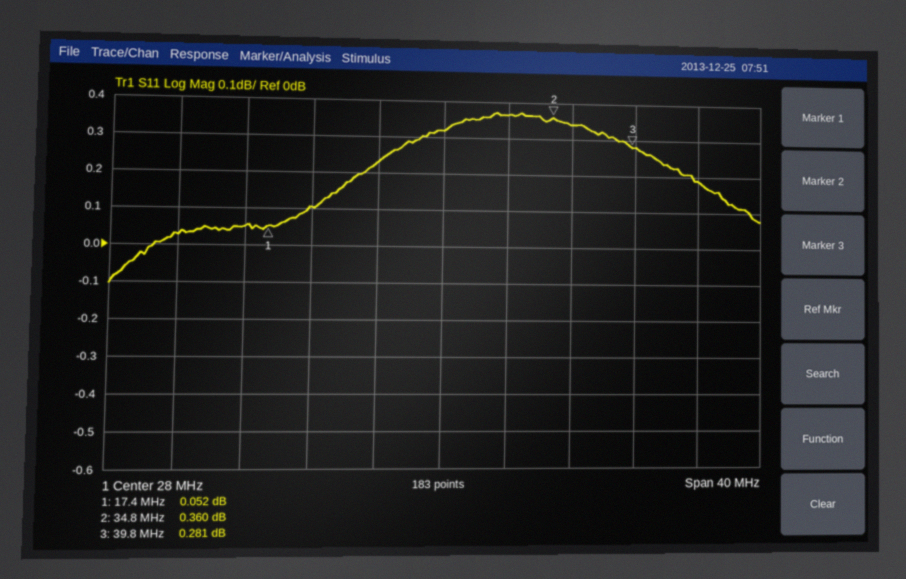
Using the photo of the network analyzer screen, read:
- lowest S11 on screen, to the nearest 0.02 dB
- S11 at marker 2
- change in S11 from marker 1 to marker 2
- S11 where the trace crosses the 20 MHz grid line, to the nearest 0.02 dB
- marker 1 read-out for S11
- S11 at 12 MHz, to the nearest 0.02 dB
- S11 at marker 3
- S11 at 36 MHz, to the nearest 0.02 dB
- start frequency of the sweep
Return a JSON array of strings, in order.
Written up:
["-0.10 dB", "0.360 dB", "0.308 dB", "0.10 dB", "0.052 dB", "0.02 dB", "0.281 dB", "0.34 dB", "8 MHz"]
